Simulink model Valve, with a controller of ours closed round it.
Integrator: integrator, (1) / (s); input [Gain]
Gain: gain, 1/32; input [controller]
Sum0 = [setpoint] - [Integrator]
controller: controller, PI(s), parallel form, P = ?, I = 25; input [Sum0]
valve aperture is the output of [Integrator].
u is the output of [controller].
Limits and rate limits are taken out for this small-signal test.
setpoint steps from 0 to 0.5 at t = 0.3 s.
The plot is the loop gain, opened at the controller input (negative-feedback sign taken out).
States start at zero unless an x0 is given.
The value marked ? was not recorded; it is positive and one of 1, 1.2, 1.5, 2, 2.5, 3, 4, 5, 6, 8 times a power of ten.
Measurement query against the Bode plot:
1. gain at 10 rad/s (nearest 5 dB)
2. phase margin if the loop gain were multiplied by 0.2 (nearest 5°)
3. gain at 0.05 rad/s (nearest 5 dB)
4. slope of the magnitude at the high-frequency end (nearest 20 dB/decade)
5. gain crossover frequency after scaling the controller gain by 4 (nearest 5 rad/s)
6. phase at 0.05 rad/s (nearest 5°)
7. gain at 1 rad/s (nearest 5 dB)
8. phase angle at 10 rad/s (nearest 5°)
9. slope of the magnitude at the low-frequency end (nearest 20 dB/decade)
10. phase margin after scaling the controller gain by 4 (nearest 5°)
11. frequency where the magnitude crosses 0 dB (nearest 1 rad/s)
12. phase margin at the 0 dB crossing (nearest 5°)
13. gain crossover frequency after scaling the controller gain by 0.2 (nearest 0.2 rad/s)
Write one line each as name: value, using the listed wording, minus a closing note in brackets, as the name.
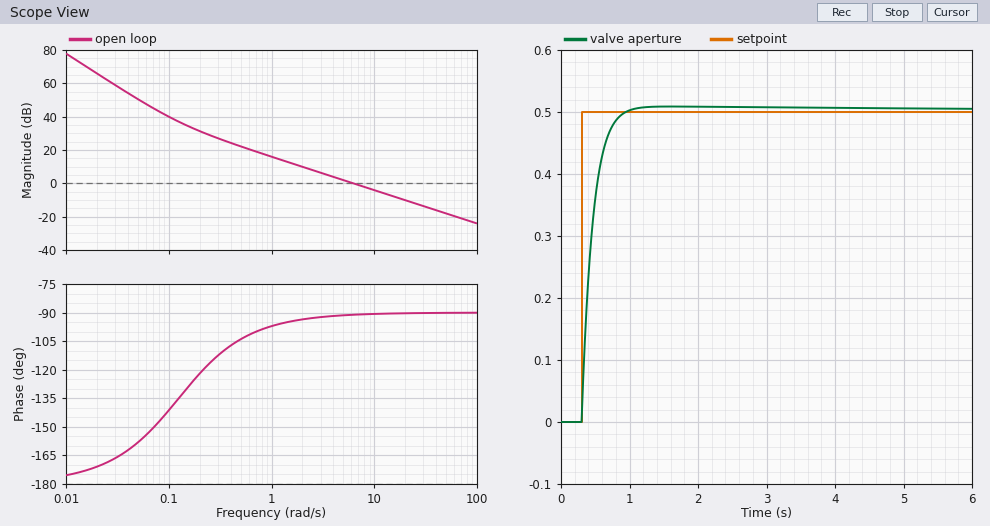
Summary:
gain at 10 rad/s: -5 dB
phase margin if the loop gain were multiplied by 0.2: 85°
gain at 0.05 rad/s: 50 dB
slope of the magnitude at the high-frequency end: -20 dB/decade
gain crossover frequency after scaling the controller gain by 4: 25 rad/s
phase at 0.05 rad/s: -160°
gain at 1 rad/s: 15 dB
phase angle at 10 rad/s: -90°
slope of the magnitude at the low-frequency end: -40 dB/decade
phase margin after scaling the controller gain by 4: 90°
frequency where the magnitude crosses 0 dB: 6 rad/s
phase margin at the 0 dB crossing: 90°
gain crossover frequency after scaling the controller gain by 0.2: 1.2 rad/s
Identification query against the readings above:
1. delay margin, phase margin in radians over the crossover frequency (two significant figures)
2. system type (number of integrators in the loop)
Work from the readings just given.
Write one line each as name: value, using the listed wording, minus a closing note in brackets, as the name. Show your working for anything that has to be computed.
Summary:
delay margin, phase margin in radians over the crossover frequency: 90 × π / 180 / 6 = 0.26 s
system type: 2
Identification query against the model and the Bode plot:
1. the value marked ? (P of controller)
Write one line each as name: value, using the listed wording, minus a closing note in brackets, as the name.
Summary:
the value marked ?: 200
